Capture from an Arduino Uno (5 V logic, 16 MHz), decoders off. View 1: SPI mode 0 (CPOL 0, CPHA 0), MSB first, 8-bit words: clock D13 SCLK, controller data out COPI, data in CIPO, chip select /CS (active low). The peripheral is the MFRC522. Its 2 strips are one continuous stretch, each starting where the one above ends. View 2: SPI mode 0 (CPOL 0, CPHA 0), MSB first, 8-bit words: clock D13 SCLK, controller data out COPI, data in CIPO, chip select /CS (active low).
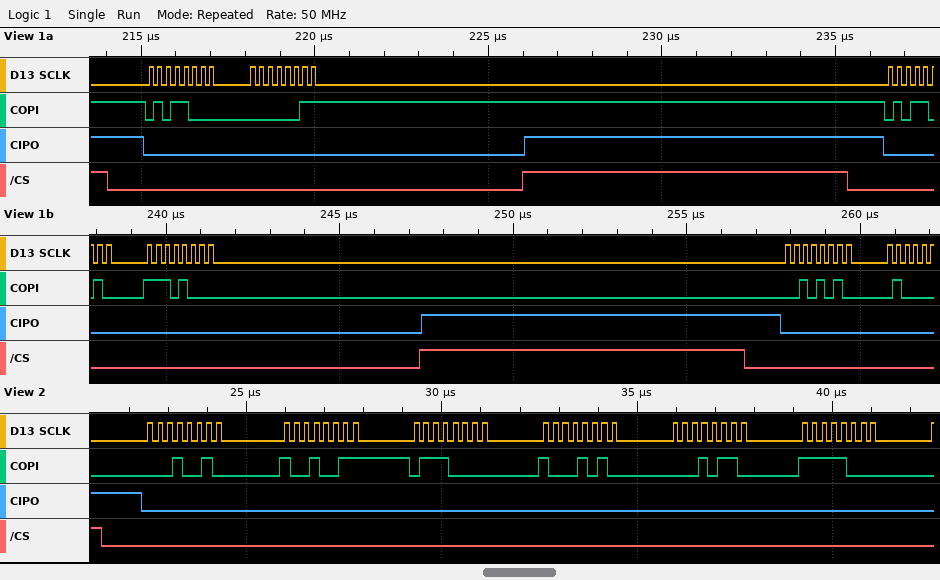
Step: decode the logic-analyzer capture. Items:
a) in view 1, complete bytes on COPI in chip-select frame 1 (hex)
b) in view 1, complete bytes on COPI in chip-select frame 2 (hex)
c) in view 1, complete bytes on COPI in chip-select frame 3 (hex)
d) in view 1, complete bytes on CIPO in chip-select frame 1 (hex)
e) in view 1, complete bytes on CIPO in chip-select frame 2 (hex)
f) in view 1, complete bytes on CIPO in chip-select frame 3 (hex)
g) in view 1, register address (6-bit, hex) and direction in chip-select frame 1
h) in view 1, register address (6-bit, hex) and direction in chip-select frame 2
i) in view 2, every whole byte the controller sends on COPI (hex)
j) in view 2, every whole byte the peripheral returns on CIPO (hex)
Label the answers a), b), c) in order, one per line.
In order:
a) 0x58 0x03
b) 0x5A 0xE8
c) 0x2A
d) 0x00 0x00
e) 0x00 0x00
f) 0x00
g) 0x2C write
h) 0x2D write
i) 0x12 0x93 0x70 0x8A 0x16 0xF8
j) 0x00 0x00 0x00 0x00 0x00 0x00
